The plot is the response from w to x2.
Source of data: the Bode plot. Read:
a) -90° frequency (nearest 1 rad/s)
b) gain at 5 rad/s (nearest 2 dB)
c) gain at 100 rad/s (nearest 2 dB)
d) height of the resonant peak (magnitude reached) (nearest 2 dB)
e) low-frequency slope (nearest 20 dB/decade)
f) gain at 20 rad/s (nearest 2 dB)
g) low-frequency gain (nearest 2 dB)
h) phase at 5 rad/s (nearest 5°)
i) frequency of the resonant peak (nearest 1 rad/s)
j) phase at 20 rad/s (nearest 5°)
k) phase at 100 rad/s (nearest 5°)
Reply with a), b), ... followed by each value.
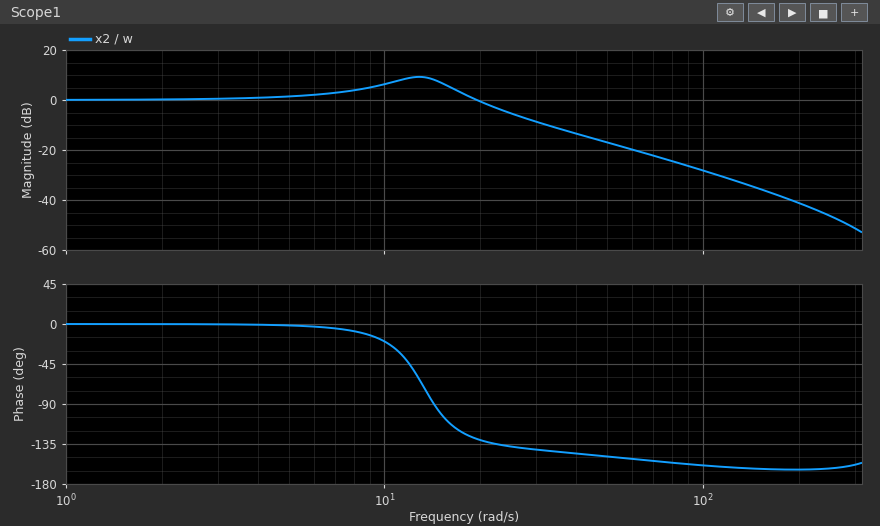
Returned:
a) 14 rad/s
b) 2 dB
c) -28 dB
d) 10 dB
e) 0 dB/decade
f) 0 dB
g) 0 dB
h) 0°
i) 13 rad/s
j) -130°
k) -160°
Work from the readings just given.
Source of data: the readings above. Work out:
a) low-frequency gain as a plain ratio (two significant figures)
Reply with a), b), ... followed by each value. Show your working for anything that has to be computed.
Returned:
a) 10^(0 / 20) = 1.0
